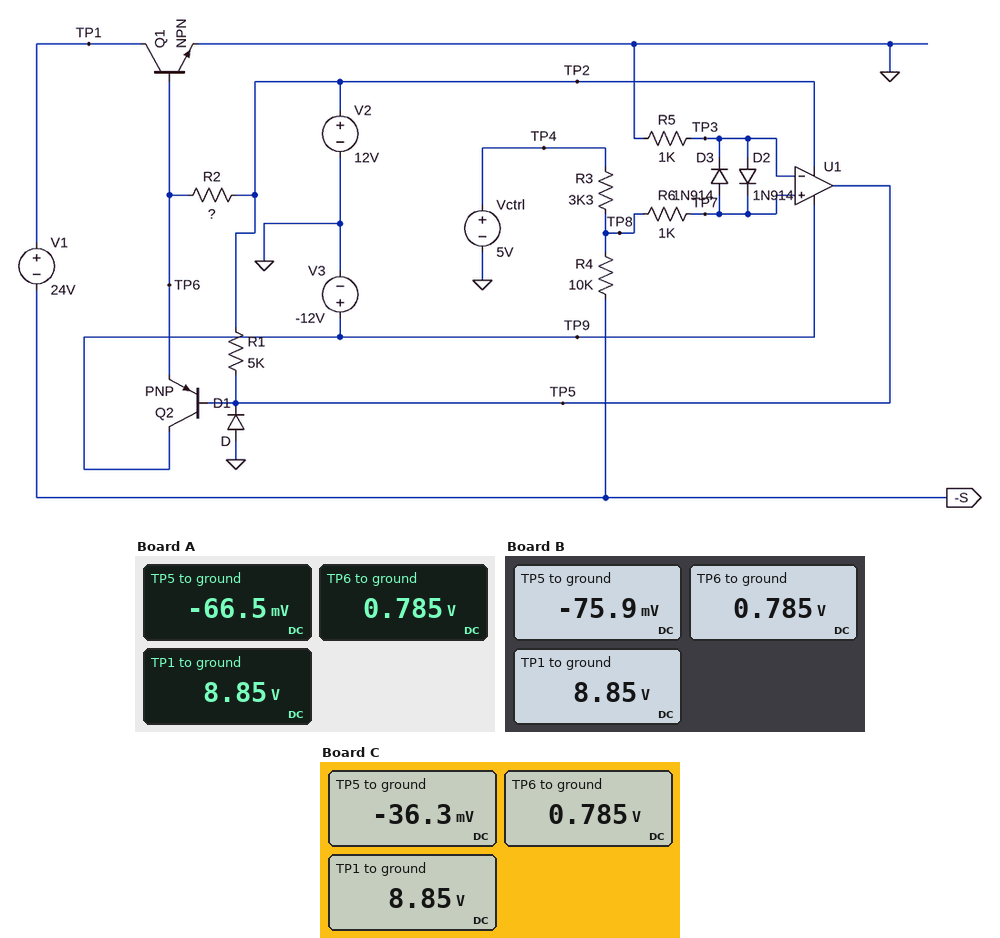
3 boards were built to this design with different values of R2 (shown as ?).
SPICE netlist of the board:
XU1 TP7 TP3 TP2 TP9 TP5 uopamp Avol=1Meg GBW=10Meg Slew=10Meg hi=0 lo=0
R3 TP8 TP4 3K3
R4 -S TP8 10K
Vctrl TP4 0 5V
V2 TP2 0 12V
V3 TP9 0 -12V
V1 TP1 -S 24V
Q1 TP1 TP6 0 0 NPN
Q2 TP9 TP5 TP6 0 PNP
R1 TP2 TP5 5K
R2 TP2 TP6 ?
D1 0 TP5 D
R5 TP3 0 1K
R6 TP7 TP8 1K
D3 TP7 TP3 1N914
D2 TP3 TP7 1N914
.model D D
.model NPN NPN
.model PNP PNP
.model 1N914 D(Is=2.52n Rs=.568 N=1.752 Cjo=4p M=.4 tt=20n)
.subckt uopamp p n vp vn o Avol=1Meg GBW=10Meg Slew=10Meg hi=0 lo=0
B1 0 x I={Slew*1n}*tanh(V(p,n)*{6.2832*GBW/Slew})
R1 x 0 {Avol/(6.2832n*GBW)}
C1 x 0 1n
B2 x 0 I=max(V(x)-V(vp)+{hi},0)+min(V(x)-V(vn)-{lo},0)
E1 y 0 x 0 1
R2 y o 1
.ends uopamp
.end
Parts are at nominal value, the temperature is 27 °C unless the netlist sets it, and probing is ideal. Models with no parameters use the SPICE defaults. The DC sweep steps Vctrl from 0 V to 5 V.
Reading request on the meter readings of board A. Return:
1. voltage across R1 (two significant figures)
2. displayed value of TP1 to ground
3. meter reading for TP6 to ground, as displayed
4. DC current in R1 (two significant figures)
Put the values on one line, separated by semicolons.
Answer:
12 V; 8.85 V; 0.785 V; 2.4 mA
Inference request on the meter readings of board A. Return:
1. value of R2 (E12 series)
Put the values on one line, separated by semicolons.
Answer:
560 Ω
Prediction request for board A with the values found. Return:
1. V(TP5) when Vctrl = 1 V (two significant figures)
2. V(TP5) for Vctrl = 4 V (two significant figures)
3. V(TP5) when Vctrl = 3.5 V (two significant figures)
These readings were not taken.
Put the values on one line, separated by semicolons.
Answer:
-110 mV; -72 mV; -76 mV
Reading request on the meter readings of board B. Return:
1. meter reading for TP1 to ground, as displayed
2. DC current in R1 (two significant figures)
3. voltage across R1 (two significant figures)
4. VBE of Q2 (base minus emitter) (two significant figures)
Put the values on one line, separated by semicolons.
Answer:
8.85 V; 2.4 mA; 12 V; -860 mV
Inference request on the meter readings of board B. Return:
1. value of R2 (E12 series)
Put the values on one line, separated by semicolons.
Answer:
390 Ω
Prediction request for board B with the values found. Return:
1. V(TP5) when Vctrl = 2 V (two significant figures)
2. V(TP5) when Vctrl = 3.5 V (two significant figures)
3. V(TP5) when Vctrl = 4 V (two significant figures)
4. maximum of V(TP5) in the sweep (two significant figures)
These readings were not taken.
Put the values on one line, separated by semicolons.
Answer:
-100 mV; -85 mV; -82 mV; -76 mV
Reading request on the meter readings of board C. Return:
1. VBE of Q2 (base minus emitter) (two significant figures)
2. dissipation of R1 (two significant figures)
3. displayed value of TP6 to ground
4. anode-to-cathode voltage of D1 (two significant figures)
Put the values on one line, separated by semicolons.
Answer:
-820 mV; 29 mW; 0.785 V; 36 mV
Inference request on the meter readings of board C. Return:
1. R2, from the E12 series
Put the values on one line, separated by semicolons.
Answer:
1.8 kΩ
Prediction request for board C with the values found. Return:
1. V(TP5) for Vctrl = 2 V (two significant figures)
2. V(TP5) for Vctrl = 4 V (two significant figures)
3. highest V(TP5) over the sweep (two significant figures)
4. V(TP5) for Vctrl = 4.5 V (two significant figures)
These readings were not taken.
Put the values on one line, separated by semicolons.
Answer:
-60 mV; -42 mV; -36 mV; -39 mV
